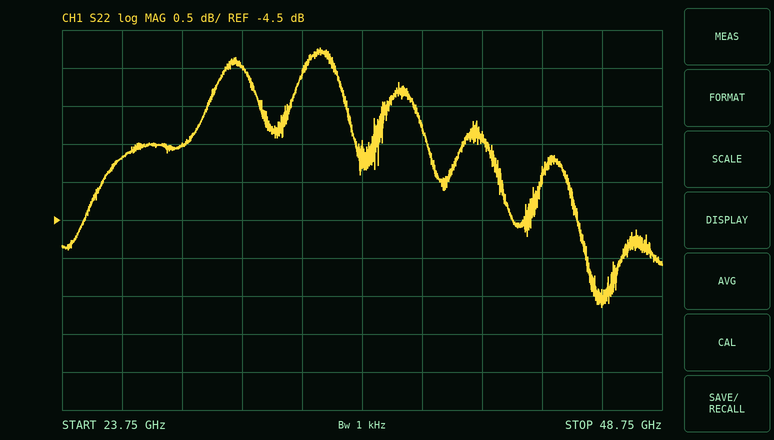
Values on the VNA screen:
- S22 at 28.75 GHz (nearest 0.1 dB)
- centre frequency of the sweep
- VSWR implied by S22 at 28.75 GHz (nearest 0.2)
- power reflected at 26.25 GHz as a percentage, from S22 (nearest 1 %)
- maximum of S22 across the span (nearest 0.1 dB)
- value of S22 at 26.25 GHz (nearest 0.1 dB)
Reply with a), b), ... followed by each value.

a) -3.5 dB
b) 36.25 GHz
c) 5.0
d) 43 %
e) -2.2 dB
f) -3.7 dB
